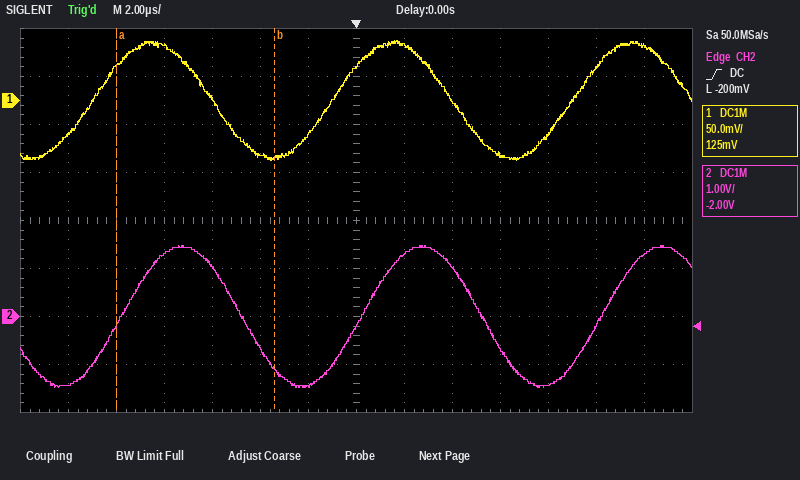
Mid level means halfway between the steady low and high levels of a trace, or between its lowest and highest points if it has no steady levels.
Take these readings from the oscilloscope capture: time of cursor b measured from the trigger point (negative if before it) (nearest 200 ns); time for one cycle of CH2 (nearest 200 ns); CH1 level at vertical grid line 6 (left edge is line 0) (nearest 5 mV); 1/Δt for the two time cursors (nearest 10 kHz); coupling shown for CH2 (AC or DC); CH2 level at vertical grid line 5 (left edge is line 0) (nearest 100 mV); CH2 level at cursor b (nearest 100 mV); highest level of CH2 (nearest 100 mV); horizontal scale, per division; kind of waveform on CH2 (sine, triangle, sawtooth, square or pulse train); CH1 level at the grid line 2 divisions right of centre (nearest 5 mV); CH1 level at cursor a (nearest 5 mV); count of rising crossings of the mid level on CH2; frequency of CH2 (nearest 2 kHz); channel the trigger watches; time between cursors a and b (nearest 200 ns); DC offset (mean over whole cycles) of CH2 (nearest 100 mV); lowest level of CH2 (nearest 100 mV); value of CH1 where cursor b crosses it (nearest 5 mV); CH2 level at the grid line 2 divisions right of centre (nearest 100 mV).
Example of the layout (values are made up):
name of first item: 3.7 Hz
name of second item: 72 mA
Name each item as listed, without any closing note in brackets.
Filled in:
time of cursor b measured from the trigger point (negative if before it): -3.4 µs
time for one cycle of CH2: 10.0 µs
CH1 level at vertical grid line 6 (left edge is line 0): -35 mV
1/Δt for the two time cursors: 150 kHz
coupling shown for CH2: DC
CH2 level at vertical grid line 5 (left edge is line 0): -700 mV
CH2 level at cursor b: -1.1 V
highest level of CH2: 1.5 V
horizontal scale, per division: 2 µs
kind of waveform on CH2: sine
CH1 level at the grid line 2 divisions right of centre: 0 mV
CH1 level at cursor a: 35 mV
count of rising crossings of the mid level on CH2: 3
frequency of CH2: 100 kHz
channel the trigger watches: CH2
time between cursors a and b: 6.6 µs
DC offset (mean over whole cycles) of CH2: 0.0 V
lowest level of CH2: -1.5 V
value of CH1 where cursor b crosses it: -60 mV
CH2 level at the grid line 2 divisions right of centre: 1.0 V
